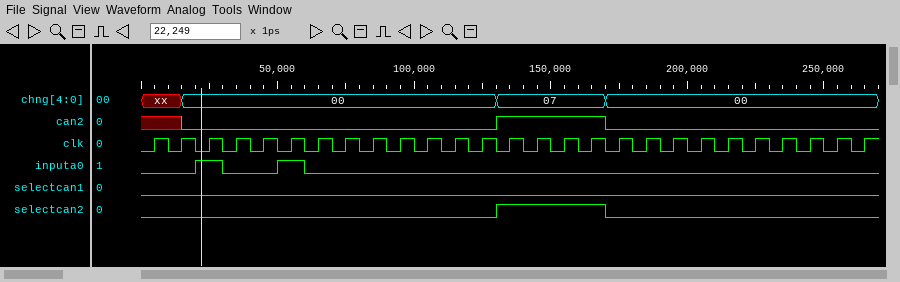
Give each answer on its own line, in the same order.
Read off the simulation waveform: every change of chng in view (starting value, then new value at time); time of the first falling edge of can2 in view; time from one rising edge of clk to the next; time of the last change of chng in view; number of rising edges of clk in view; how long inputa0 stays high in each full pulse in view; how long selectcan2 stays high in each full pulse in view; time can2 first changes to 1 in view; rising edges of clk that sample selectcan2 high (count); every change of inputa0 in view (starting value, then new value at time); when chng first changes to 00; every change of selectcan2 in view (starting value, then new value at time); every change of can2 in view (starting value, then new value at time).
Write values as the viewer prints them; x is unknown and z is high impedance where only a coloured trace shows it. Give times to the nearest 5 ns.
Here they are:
xx, 00 at 15 ns, 07 at 130 ns, 00 at 170 ns
170 ns
10 ns
170 ns
27
10 ns, 10 ns
40 ns
130 ns
4
0, 1 at 20 ns, 0 at 30 ns, 1 at 50 ns, 0 at 60 ns
15 ns
0, 1 at 130 ns, 0 at 170 ns
x, 0 at 15 ns, 1 at 130 ns, 0 at 170 ns
